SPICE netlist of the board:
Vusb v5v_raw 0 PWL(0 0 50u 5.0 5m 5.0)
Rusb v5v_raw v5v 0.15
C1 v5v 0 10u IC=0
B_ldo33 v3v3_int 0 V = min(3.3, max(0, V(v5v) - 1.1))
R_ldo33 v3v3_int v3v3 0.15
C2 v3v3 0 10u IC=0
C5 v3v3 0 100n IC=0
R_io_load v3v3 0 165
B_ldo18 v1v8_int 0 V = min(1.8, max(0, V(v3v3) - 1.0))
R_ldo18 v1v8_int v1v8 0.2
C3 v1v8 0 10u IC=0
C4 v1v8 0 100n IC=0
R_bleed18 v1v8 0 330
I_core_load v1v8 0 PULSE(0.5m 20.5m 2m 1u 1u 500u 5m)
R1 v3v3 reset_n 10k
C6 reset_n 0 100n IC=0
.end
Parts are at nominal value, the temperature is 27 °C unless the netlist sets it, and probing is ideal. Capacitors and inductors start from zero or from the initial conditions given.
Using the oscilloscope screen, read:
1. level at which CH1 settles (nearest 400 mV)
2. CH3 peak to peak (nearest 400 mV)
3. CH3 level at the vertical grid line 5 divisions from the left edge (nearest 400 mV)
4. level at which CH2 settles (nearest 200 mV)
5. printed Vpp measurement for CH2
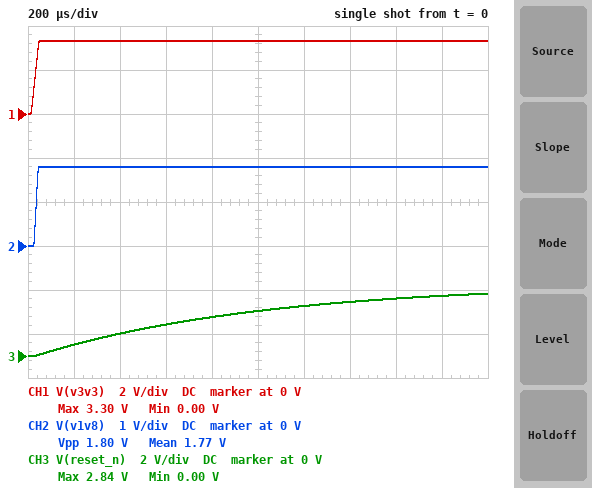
3.2 V
2.8 V
2.0 V
1.8 V
1.80 V
